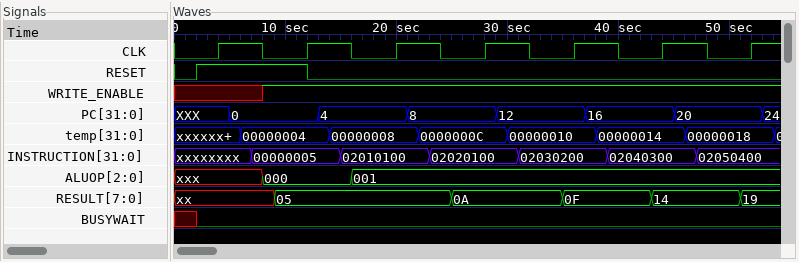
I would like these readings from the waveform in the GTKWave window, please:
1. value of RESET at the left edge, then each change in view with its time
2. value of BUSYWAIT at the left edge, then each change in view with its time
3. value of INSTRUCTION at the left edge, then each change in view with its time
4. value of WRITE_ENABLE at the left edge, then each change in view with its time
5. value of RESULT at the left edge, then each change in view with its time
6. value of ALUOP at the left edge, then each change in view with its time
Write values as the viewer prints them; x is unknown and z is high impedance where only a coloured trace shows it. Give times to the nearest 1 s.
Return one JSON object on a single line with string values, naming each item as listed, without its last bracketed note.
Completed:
{"value of RESET at the left edge, then each change in view with its time": "0, 1 at 2 s, 0 at 12 s", "value of BUSYWAIT at the left edge, then each change in view with its time": "x, 0 at 2 s", "value of INSTRUCTION at the left edge, then each change in view with its time": "xxxxxxxx, 00000005 at 7 s, 02010100 at 15 s, 02020100 at 23 s, 02030200 at 31 s, 02040300 at 39 s, 02050400 at 47 s", "value of WRITE_ENABLE at the left edge, then each change in view with its time": "x, 1 at 8 s", "value of RESULT at the left edge, then each change in view with its time": "xx, 05 at 9 s, 0A at 25 s, 0F at 35 s, 14 at 43 s, 19 at 51 s", "value of ALUOP at the left edge, then each change in view with its time": "xxx, 000 at 8 s, 001 at 16 s"}
